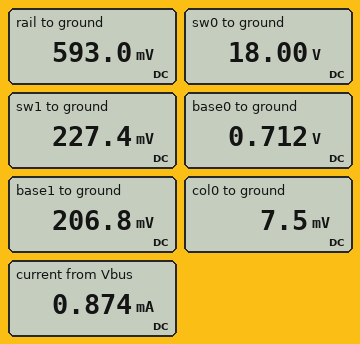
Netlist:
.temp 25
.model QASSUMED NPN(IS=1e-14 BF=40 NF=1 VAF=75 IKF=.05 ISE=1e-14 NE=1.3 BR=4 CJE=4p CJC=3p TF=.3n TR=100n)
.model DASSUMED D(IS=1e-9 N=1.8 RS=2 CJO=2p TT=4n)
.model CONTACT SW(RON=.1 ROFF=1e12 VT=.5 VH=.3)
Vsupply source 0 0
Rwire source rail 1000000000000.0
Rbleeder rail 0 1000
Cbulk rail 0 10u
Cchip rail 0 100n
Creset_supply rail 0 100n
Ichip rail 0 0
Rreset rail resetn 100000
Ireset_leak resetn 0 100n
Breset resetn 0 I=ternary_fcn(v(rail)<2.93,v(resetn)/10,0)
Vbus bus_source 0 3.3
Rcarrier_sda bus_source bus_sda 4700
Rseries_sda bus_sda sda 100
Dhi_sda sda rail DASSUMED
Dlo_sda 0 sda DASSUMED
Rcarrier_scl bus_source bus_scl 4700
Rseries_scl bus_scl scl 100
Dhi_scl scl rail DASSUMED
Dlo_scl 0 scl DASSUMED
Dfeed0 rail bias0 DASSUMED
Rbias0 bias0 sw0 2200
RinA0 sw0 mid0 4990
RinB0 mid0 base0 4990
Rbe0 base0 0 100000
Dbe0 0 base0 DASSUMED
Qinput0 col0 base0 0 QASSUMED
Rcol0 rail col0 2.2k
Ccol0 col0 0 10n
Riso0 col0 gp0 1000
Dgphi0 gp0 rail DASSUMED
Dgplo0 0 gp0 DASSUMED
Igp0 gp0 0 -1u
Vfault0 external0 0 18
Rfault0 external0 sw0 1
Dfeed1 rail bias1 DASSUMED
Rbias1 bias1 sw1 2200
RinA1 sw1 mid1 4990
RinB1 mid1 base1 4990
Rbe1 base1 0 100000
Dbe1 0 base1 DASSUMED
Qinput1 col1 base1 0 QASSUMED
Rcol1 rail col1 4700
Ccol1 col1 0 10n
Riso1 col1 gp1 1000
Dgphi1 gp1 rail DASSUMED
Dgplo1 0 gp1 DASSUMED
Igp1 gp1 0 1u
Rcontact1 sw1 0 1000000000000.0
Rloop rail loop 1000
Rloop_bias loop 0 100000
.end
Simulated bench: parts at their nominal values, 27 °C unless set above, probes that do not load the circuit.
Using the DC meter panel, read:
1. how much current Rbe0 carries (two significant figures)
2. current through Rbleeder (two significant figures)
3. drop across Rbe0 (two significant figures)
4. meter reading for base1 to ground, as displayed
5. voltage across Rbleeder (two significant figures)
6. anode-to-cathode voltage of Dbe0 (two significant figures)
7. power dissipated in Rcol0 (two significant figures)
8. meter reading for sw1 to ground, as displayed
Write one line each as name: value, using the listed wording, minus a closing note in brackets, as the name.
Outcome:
how much current Rbe0 carries: 7.1 µA
current through Rbleeder: 590 µA
drop across Rbe0: 710 mV
meter reading for base1 to ground, as displayed: 206.8 mV
voltage across Rbleeder: 590 mV
anode-to-cathode voltage of Dbe0: -710 mV
power dissipated in Rcol0: 160 µW
meter reading for sw1 to ground, as displayed: 227.4 mV
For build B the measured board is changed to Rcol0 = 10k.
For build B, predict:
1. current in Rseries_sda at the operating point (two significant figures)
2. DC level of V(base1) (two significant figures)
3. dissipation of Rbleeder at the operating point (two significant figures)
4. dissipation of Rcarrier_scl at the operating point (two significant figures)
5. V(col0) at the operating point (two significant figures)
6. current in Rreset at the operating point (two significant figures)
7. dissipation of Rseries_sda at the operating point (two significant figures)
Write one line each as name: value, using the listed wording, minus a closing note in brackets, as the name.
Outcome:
current in Rseries_sda at the operating point: 410 µA
DC level of V(base1): 310 mV
dissipation of Rbleeder at the operating point: 530 µW
dissipation of Rcarrier_scl at the operating point: 790 µW
V(col0) at the operating point: 6.8 mV
current in Rreset at the operating point: 7.3 µA
dissipation of Rseries_sda at the operating point: 17 µW
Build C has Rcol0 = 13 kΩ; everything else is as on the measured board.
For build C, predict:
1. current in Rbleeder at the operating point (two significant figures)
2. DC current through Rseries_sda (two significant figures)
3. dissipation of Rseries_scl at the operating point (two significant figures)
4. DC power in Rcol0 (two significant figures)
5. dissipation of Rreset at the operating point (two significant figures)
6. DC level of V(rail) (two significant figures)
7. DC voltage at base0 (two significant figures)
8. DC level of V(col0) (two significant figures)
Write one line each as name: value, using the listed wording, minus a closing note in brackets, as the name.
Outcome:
current in Rbleeder at the operating point: 740 µA
DC current through Rseries_sda: 410 µA
dissipation of Rseries_scl at the operating point: 17 µW
DC power in Rcol0: 41 µW
dissipation of Rreset at the operating point: 5.5 µW
DC level of V(rail): 740 mV
DC voltage at base0: 710 mV
DC level of V(col0): 6.7 mV
